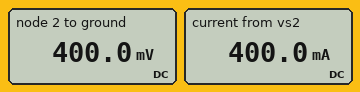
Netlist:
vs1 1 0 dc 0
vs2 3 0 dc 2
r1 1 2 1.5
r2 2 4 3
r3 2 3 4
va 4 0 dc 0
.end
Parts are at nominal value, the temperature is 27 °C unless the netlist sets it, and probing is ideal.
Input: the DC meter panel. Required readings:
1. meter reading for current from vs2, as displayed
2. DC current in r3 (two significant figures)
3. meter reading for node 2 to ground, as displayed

400.0 mA
400 mA
400.0 mV
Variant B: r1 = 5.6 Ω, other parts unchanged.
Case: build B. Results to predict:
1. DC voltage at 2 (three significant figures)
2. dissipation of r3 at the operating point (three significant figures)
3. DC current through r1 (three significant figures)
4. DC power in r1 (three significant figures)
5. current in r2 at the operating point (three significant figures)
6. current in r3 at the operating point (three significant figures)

656 mV
451 mW
117 mA
76.9 mW
219 mA
336 mA
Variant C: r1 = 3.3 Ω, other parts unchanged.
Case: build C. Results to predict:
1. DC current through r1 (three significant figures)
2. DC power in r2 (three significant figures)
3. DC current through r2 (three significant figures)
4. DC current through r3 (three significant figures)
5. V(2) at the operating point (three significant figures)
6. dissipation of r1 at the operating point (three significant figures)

171 mA
106 mW
188 mA
359 mA
564 mV
96.4 mW
